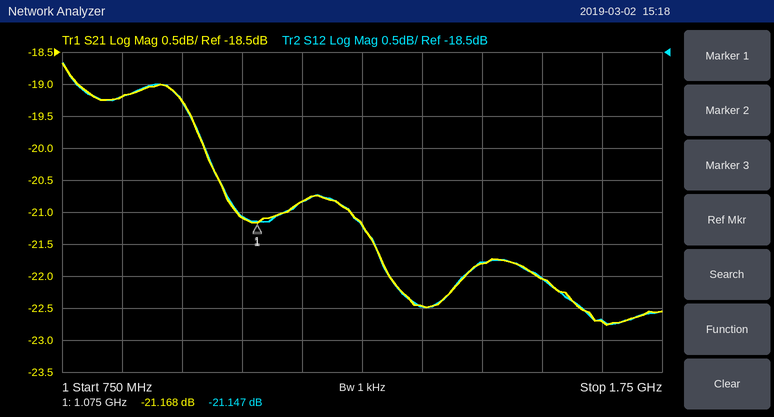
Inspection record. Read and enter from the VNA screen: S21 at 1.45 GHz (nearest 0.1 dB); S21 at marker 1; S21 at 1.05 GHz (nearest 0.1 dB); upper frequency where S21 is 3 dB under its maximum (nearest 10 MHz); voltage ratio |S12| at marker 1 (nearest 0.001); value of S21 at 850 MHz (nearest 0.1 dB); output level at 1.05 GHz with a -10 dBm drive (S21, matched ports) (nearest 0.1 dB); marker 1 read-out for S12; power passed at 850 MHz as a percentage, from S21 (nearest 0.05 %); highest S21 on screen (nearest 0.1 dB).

-21.8 dB
-21.168 dB
-21.1 dB
1.28 GHz
0.088
-19.2 dB
-31.1 dBm
-21.147 dB
1.20 %
-18.7 dB
